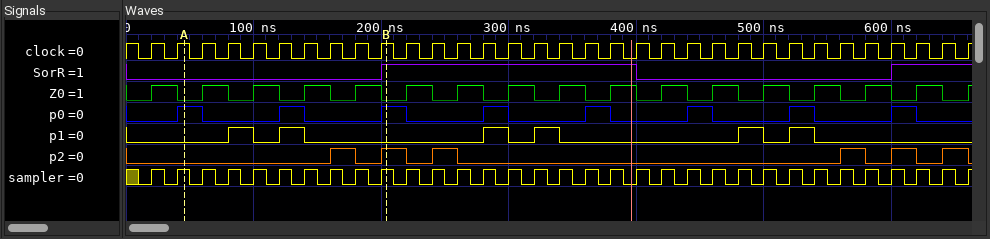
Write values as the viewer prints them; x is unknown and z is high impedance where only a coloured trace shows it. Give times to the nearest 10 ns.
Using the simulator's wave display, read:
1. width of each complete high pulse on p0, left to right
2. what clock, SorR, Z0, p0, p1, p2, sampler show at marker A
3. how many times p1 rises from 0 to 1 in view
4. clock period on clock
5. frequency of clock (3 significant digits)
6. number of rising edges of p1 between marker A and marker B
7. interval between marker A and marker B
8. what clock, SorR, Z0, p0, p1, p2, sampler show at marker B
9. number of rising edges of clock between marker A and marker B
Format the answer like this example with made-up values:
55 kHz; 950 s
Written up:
20 ns, 20 ns, 20 ns, 20 ns, 20 ns, 20 ns, 20 ns, 20 ns; clock=1, SorR=0, Z0=0, p0=1, p1=0, p2=0, sampler=1; 6; 20 ns; 50.0 MHz; 2; 160 ns; clock=1, SorR=1, Z0=0, p0=1, p1=0, p2=1, sampler=1; 8
